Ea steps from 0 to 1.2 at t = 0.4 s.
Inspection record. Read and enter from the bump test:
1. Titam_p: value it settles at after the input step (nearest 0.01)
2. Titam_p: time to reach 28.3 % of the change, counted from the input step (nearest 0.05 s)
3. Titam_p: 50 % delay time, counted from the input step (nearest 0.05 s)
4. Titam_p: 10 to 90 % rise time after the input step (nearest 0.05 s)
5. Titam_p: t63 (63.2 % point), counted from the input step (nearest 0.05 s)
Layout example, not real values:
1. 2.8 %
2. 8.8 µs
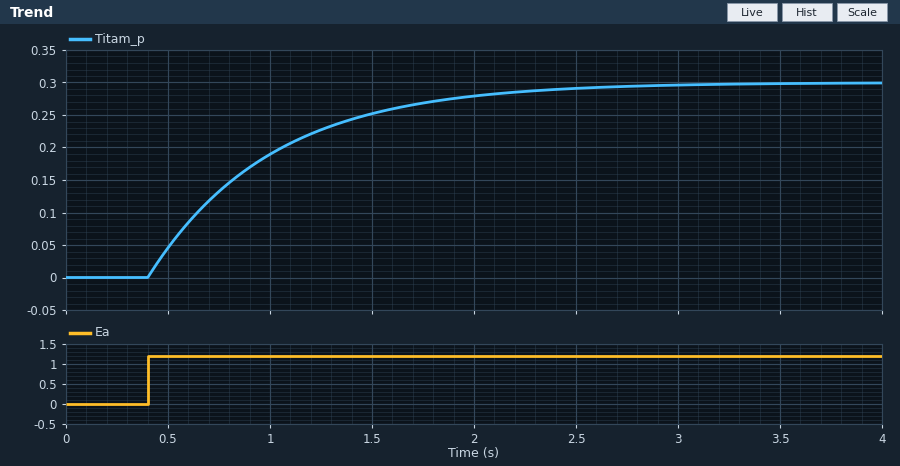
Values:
1. 0.30
2. 0.20 s
3. 0.40 s
4. 1.30 s
5. 0.60 s
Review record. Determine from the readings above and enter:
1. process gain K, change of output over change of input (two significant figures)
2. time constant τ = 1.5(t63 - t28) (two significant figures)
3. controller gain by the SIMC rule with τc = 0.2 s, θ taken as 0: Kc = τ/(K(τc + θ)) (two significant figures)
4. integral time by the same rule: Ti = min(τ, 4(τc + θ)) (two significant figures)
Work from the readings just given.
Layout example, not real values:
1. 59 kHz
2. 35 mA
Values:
1. 0.25
2. 0.60 s
3. 12
4. 0.60 s
